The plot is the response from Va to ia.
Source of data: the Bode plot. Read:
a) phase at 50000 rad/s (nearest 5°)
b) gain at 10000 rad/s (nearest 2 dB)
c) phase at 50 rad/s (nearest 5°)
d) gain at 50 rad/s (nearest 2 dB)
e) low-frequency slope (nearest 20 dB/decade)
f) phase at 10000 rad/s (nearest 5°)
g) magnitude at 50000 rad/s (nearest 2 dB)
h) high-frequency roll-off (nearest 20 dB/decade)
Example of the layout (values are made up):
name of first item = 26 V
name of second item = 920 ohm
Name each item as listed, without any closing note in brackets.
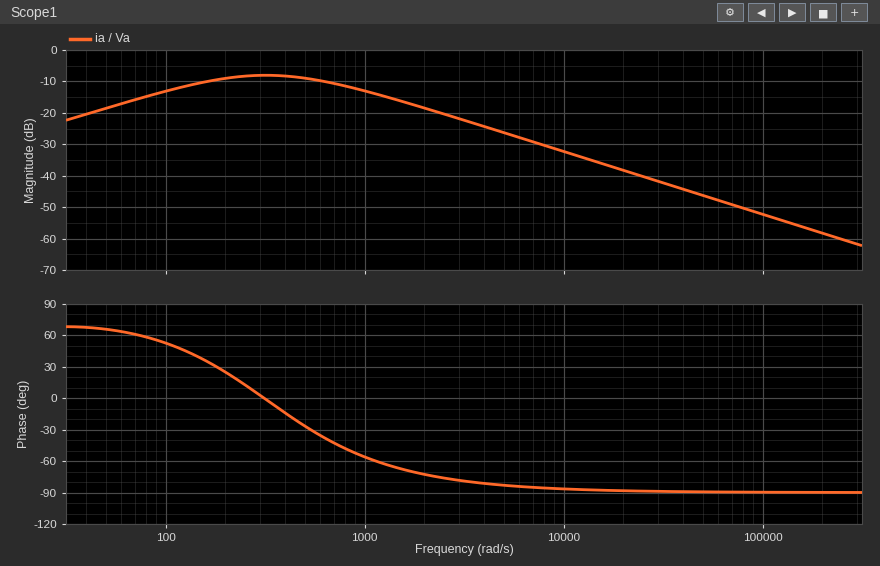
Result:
phase at 50000 rad/s = -90°
gain at 10000 rad/s = -32 dB
phase at 50 rad/s = 65°
gain at 50 rad/s = -18 dB
low-frequency slope = 20 dB/decade
phase at 10000 rad/s = -85°
magnitude at 50000 rad/s = -46 dB
high-frequency roll-off = -20 dB/decade
